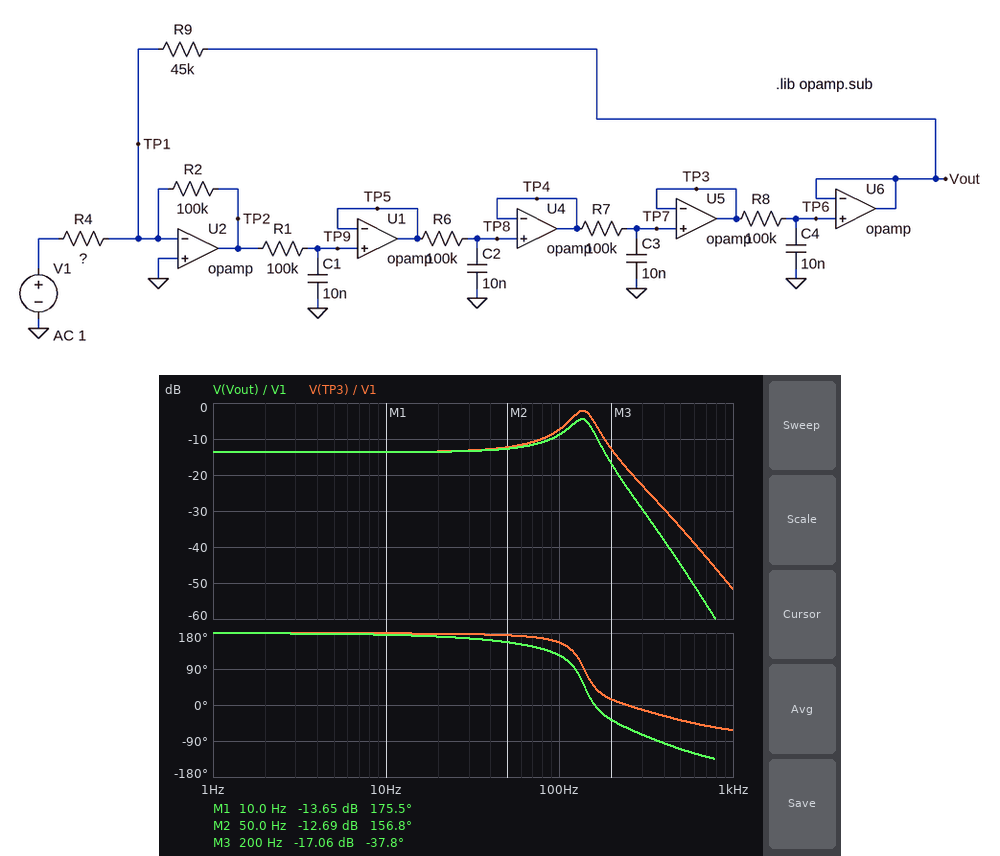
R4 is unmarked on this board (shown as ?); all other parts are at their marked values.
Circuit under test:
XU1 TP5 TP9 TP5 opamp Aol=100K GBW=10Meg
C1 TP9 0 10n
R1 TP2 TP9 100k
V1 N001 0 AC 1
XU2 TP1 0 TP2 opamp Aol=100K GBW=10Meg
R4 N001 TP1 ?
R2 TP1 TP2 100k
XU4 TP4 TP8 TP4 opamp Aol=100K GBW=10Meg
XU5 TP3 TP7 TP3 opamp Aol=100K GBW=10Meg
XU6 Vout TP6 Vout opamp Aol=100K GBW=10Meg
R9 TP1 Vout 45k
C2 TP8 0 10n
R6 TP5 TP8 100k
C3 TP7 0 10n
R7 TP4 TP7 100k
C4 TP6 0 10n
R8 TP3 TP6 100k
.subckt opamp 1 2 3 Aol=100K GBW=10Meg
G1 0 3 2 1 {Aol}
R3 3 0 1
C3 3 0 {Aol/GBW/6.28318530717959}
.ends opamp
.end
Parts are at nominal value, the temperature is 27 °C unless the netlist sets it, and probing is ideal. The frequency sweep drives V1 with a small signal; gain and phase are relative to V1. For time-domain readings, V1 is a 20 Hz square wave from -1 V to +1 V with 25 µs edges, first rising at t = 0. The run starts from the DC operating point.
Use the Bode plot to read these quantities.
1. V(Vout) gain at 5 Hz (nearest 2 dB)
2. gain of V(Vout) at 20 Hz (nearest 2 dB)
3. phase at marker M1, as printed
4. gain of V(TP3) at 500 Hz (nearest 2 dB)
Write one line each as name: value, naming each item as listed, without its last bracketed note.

V(Vout) gain at 5 Hz: -14 dB
gain of V(Vout) at 20 Hz: -14 dB
phase at marker M1, as printed: 175.5 deg
gain of V(TP3) at 500 Hz: -34 dB
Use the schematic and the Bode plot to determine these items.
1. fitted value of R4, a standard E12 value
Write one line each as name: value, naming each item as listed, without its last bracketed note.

fitted value of R4, a standard E12 value: 150 kΩ
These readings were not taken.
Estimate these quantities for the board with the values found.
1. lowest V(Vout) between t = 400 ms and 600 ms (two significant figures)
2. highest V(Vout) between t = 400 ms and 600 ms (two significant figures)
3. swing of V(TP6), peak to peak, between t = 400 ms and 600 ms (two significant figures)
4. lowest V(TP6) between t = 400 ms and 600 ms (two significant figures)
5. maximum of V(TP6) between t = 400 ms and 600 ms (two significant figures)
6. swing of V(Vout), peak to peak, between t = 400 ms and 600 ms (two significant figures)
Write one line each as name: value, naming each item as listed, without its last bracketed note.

lowest V(Vout) between t = 400 ms and 600 ms: -440 mV
highest V(Vout) between t = 400 ms and 600 ms: 440 mV
swing of V(TP6), peak to peak, between t = 400 ms and 600 ms: 870 mV
lowest V(TP6) between t = 400 ms and 600 ms: -440 mV
maximum of V(TP6) between t = 400 ms and 600 ms: 440 mV
swing of V(Vout), peak to peak, between t = 400 ms and 600 ms: 870 mV
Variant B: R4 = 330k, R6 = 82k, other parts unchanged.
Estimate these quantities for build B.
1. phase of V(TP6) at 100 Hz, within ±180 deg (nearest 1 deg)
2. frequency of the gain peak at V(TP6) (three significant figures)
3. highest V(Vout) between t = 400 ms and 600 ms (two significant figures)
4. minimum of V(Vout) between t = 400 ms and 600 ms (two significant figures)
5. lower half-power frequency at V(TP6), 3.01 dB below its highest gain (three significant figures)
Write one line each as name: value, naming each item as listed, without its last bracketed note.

phase of V(TP6) at 100 Hz, within ±180 deg: 128 deg
frequency of the gain peak at V(TP6): 141 Hz
highest V(Vout) between t = 400 ms and 600 ms: 200 mV
minimum of V(Vout) between t = 400 ms and 600 ms: -200 mV
lower half-power frequency at V(TP6), 3.01 dB below its highest gain: 114 Hz
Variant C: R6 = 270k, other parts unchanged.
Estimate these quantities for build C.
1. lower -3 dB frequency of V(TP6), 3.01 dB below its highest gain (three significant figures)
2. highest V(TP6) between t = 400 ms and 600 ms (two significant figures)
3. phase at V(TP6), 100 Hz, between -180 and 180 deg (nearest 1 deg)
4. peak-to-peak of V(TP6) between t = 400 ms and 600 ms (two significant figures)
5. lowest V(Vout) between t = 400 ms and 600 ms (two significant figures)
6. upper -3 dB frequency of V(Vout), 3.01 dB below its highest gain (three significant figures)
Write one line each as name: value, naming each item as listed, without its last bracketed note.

lower -3 dB frequency of V(TP6), 3.01 dB below its highest gain: 68.6 Hz
highest V(TP6) between t = 400 ms and 600 ms: 400 mV
phase at V(TP6), 100 Hz, between -180 and 180 deg: 61 deg
peak-to-peak of V(TP6) between t = 400 ms and 600 ms: 790 mV
lowest V(Vout) between t = 400 ms and 600 ms: -400 mV
upper -3 dB frequency of V(Vout), 3.01 dB below its highest gain: 118 Hz
